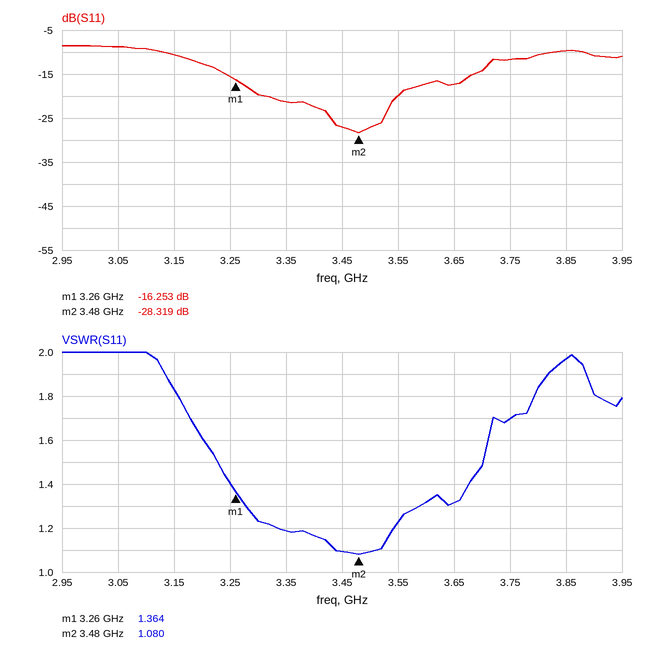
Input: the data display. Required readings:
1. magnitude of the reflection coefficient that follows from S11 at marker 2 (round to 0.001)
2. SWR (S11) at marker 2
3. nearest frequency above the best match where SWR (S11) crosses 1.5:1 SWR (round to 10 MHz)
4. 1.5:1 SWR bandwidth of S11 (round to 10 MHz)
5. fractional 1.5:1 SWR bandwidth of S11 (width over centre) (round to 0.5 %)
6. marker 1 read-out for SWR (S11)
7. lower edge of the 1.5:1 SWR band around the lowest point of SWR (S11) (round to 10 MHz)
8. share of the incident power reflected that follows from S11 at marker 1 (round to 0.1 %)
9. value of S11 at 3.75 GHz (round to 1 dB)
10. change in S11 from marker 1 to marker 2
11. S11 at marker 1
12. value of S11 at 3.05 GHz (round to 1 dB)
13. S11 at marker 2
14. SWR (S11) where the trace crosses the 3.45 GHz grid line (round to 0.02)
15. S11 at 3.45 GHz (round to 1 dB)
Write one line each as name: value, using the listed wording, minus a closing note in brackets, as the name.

magnitude of the reflection coefficient that follows from S11 at marker 2: 0.038
SWR (S11) at marker 2: 1.080
nearest frequency above the best match where SWR (S11) crosses 1.5:1 SWR: 3.70 GHz
1.5:1 SWR bandwidth of S11: 470 MHz
fractional 1.5:1 SWR bandwidth of S11 (width over centre): 13.5 %
marker 1 read-out for SWR: 1.364
lower edge of the 1.5:1 SWR band around the lowest point of SWR (S11): 3.23 GHz
share of the incident power reflected that follows from S11 at marker 1: 2.4 %
value of S11 at 3.75 GHz: -12 dB
change in S11 from marker 1 to marker 2: -12.066 dB
S11 at marker 1: -16.253 dB
value of S11 at 3.05 GHz: -9 dB
S11 at marker 2: -28.319 dB
SWR (S11) where the trace crosses the 3.45 GHz grid line: 1.10
S11 at 3.45 GHz: -27 dB
